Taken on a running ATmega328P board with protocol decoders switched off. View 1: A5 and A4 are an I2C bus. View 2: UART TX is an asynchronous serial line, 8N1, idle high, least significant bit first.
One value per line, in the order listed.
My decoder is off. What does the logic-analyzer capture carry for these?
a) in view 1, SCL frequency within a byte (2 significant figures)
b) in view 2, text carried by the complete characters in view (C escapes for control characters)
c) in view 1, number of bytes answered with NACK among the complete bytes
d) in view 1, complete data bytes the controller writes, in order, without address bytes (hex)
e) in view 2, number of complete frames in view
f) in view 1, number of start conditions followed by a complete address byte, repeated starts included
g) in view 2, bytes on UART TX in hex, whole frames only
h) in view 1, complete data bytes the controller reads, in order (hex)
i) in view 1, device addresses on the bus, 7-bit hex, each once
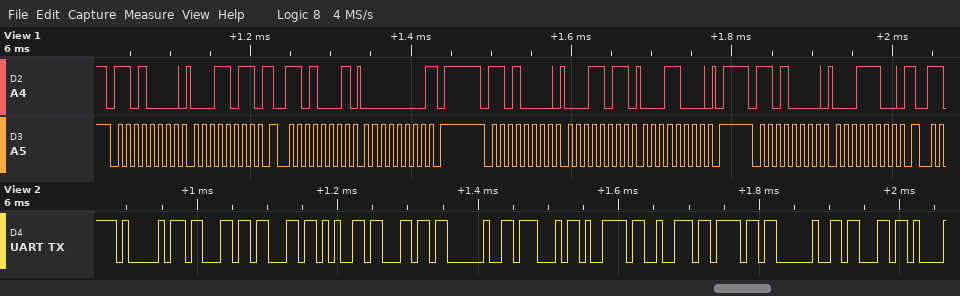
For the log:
100 kHz
"Accel Gyro c"
1
1B 1B 18 1C
12
4
41 63 63 65 6C 20 47 79 72 6F 20 63
00
0x68
